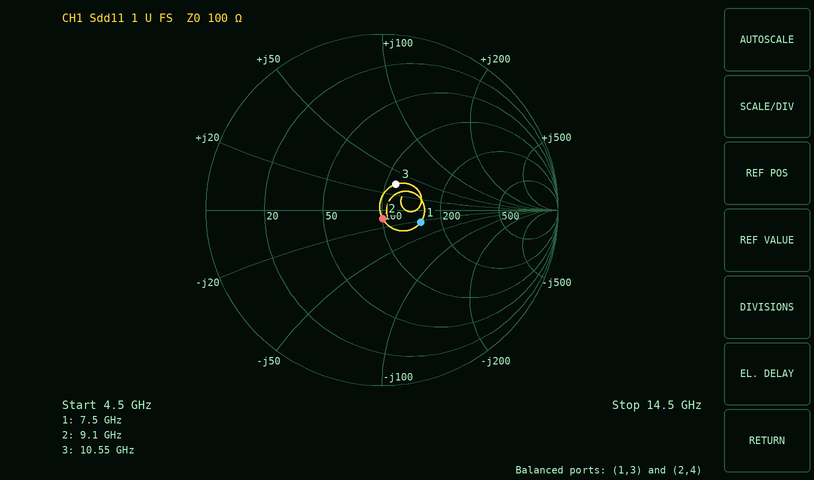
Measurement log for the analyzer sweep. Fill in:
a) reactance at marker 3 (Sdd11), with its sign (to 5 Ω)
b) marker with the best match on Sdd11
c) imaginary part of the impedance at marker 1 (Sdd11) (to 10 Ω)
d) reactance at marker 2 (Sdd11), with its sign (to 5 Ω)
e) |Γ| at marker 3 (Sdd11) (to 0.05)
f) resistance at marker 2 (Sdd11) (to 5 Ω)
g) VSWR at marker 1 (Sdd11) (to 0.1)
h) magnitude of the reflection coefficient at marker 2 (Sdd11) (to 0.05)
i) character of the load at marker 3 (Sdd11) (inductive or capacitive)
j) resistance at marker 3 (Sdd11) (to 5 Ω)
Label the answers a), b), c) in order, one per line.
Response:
a) +35 Ω
b) marker 2
c) -20 Ω
d) -10 Ω
e) 0.15
f) 100 Ω
g) 1.6
h) 0.05
i) inductive
j) 110 Ω
